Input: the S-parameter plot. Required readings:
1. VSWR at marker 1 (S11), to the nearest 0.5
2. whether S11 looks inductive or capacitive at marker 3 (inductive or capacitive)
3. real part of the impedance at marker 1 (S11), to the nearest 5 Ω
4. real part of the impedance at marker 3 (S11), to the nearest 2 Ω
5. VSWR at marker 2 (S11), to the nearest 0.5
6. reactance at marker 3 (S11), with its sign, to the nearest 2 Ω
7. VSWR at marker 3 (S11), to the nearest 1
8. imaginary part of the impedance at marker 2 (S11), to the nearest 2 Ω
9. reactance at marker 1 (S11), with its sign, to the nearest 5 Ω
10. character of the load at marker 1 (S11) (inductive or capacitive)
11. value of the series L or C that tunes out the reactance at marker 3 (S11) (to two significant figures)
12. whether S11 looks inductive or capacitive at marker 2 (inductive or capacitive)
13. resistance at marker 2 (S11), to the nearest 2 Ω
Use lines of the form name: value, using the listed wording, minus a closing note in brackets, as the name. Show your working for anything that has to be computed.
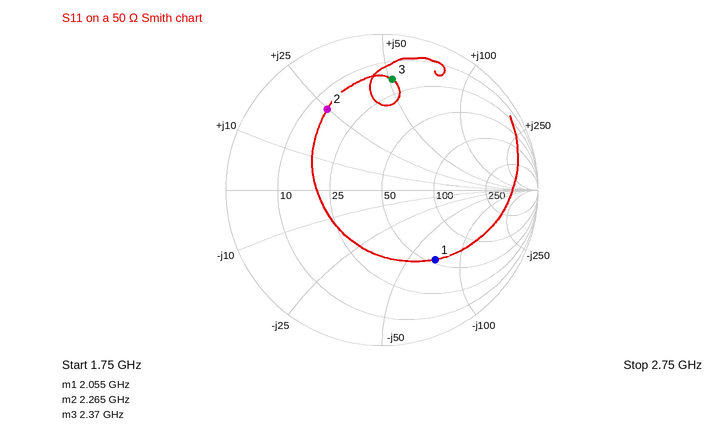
VSWR at marker 1 (S11), to the nearest 0.5: 3.5
whether S11 looks inductive or capacitive at marker 3: inductive
real part of the impedance at marker 1 (S11), to the nearest 5 Ω: 55 Ω
real part of the impedance at marker 3 (S11), to the nearest 2 Ω: 18 Ω
VSWR at marker 2 (S11), to the nearest 0.5: 4.5
reactance at marker 3 (S11), with its sign, to the nearest 2 Ω: +52 Ω
VSWR at marker 3 (S11), to the nearest 1: 6
imaginary part of the impedance at marker 2 (S11), to the nearest 2 Ω: +24 Ω
reactance at marker 1 (S11), with its sign, to the nearest 5 Ω: -70 Ω
character of the load at marker 1 (S11): capacitive
value of the series L or C that tunes out the reactance at marker 3 (S11): C = 1/(2π × 2.37 GHz × 52 Ω) ≈ 1.3 pF
whether S11 looks inductive or capacitive at marker 2: inductive
resistance at marker 2 (S11), to the nearest 2 Ω: 14 Ω
